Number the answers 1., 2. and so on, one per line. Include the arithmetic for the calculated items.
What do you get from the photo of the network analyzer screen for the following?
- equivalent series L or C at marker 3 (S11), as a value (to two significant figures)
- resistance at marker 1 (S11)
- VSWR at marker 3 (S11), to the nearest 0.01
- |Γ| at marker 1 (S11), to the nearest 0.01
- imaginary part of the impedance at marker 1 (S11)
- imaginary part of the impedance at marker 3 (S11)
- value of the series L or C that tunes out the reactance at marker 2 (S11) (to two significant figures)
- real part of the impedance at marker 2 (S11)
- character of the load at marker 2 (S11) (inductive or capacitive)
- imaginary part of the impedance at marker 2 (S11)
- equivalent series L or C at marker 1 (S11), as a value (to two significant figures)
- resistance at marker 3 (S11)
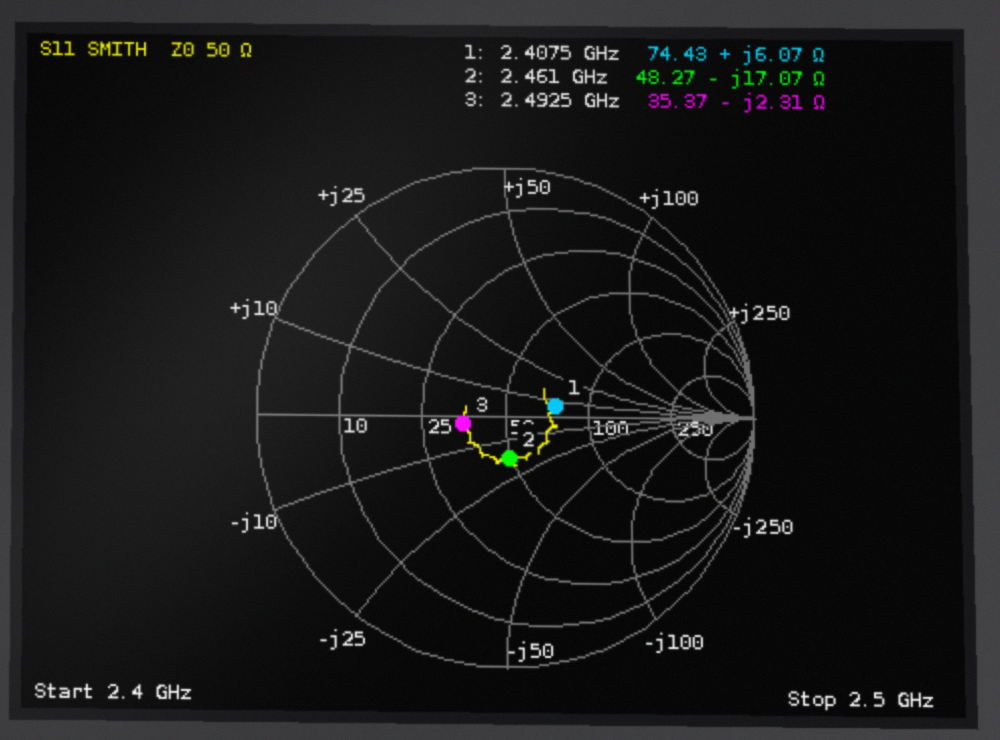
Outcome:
1. C = 1/(2π × 2.4925 GHz × 2.31 Ω) ≈ 28 pF
2. 74.43 Ω
3. 1.42
4. 0.20
5. +6.07 Ω
6. -2.31 Ω
7. L = 17.07 Ω/(2π × 2.461 GHz) ≈ 1.1 nH
8. 48.27 Ω
9. capacitive
10. -17.07 Ω
11. L = 6.07 Ω/(2π × 2.4075 GHz) ≈ 401 pH, so 400 pH to two significant figures
12. 35.37 Ω
